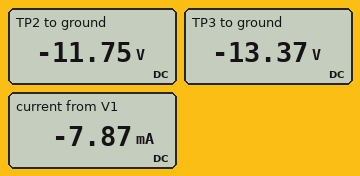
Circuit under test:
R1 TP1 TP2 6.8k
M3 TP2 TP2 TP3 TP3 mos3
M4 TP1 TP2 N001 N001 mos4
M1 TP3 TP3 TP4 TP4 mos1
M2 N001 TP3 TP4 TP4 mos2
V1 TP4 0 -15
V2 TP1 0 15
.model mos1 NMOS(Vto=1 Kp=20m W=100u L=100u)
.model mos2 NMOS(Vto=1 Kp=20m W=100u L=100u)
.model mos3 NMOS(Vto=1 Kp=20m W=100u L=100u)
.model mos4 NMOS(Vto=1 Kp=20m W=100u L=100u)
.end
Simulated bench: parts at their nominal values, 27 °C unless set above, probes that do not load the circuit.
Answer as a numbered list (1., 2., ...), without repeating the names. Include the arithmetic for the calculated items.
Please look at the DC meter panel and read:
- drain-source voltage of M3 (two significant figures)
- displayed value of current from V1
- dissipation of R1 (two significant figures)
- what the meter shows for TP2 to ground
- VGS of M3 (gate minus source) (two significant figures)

1. -11.75 V - (-13.37 V) = 1.6 V
2. -7.87 mA
3. (15 V - (-11.75 V))^2 / 6.8 kΩ = 110 mW
4. -11.75 V
5. -11.75 V - (-13.37 V) = 1.6 V
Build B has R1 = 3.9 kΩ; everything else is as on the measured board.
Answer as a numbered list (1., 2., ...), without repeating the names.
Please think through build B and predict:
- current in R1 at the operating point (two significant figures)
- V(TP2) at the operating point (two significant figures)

1. 6.8 mA
2. -11 V
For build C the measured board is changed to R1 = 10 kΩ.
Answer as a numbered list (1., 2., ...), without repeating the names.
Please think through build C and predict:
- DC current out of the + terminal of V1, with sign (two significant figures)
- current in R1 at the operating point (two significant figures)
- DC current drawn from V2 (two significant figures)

1. -5.4 mA
2. 2.7 mA
3. 5.4 mA
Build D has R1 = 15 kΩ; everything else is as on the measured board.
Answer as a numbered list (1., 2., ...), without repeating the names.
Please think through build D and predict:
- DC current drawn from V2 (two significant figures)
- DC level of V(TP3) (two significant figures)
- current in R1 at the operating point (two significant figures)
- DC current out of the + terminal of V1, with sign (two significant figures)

1. 3.6 mA
2. -14 V
3. 1.8 mA
4. -3.6 mA
